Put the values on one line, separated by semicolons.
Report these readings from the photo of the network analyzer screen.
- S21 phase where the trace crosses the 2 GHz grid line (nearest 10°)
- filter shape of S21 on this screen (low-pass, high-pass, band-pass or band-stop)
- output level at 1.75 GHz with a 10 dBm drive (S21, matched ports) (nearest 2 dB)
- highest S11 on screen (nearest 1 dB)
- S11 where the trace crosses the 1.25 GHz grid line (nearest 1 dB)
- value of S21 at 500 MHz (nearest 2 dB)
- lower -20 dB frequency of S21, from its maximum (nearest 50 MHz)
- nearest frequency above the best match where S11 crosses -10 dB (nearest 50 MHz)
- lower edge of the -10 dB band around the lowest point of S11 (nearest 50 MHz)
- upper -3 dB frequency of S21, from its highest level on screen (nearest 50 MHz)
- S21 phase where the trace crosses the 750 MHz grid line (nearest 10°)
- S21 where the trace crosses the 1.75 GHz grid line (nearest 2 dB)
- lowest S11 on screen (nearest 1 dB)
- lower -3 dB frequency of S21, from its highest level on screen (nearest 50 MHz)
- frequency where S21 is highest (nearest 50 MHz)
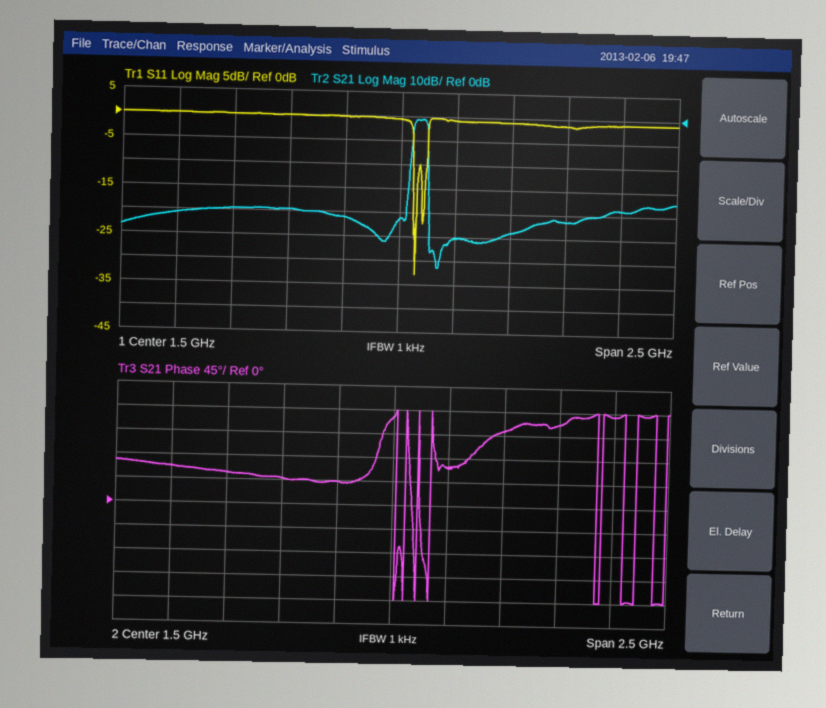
140°; band-pass; -40 dBm; 0 dB; 0 dB; -42 dB; 1.55 GHz; 1.60 GHz; 1.55 GHz; 1.60 GHz; 60°; -50 dB; -33 dB; 1.55 GHz; 1.60 GHz
